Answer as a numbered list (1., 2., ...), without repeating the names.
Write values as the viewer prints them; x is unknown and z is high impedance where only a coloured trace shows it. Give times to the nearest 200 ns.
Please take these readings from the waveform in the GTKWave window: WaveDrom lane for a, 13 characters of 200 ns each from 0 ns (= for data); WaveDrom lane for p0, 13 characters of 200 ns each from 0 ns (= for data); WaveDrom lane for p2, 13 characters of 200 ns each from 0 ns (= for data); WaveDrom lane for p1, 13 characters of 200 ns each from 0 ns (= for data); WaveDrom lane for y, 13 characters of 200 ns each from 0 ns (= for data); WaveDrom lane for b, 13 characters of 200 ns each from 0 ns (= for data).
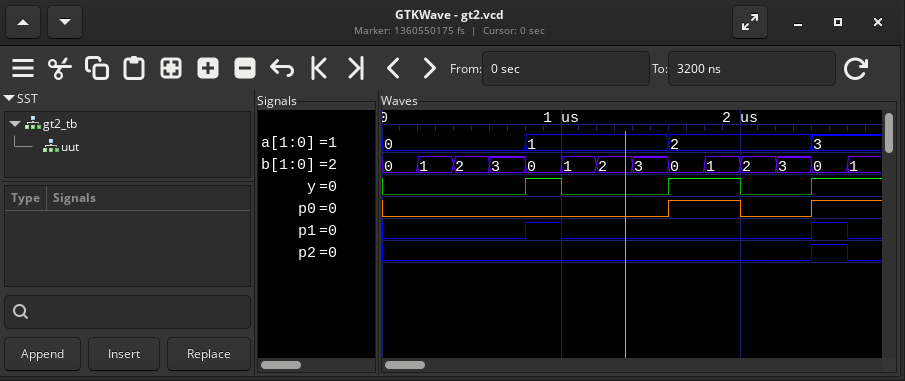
1. {name: 'a', wave: '=...=...=...=', data: '0 1 2 3'}
2. {name: 'p0', wave: '0.......1.0.1'}
3. {name: 'p2', wave: '0...........1'}
4. {name: 'p1', wave: '0...10......1'}
5. {name: 'y', wave: '0...10..1.0.1'}
6. {name: 'b', wave: '=============', data: '0 1 2 3 0 1 2 3 0 1 2 3 0'}
